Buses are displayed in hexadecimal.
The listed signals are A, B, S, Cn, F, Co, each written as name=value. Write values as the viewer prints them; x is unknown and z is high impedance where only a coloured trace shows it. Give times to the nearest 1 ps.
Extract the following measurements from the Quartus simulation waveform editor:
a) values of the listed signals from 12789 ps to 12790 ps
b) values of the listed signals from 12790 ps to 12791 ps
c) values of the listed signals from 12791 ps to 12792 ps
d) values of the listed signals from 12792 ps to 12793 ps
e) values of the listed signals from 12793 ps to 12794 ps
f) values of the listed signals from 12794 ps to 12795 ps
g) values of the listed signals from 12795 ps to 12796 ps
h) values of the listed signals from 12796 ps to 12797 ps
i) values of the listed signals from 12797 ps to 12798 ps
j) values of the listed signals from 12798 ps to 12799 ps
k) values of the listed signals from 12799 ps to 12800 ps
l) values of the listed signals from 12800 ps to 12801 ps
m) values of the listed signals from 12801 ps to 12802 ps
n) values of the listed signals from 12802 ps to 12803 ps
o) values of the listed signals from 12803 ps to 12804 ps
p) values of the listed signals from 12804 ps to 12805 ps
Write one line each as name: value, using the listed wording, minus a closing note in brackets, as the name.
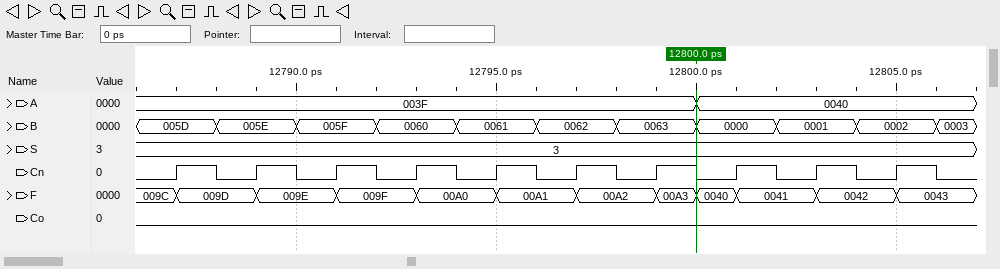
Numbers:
values of the listed signals from 12789 ps to 12790 ps: A=003F, B=005E, S=3, Cn=1, F=009E, Co=0
values of the listed signals from 12790 ps to 12791 ps: A=003F, B=005F, S=3, Cn=0, F=009E, Co=0
values of the listed signals from 12791 ps to 12792 ps: A=003F, B=005F, S=3, Cn=1, F=009F, Co=0
values of the listed signals from 12792 ps to 12793 ps: A=003F, B=0060, S=3, Cn=0, F=009F, Co=0
values of the listed signals from 12793 ps to 12794 ps: A=003F, B=0060, S=3, Cn=1, F=00A0, Co=0
values of the listed signals from 12794 ps to 12795 ps: A=003F, B=0061, S=3, Cn=0, F=00A0, Co=0
values of the listed signals from 12795 ps to 12796 ps: A=003F, B=0061, S=3, Cn=1, F=00A1, Co=0
values of the listed signals from 12796 ps to 12797 ps: A=003F, B=0062, S=3, Cn=0, F=00A1, Co=0
values of the listed signals from 12797 ps to 12798 ps: A=003F, B=0062, S=3, Cn=1, F=00A2, Co=0
values of the listed signals from 12798 ps to 12799 ps: A=003F, B=0063, S=3, Cn=0, F=00A2, Co=0
values of the listed signals from 12799 ps to 12800 ps: A=003F, B=0063, S=3, Cn=1, F=00A3, Co=0
values of the listed signals from 12800 ps to 12801 ps: A=0040, B=0000, S=3, Cn=0, F=0040, Co=0
values of the listed signals from 12801 ps to 12802 ps: A=0040, B=0000, S=3, Cn=1, F=0041, Co=0
values of the listed signals from 12802 ps to 12803 ps: A=0040, B=0001, S=3, Cn=0, F=0041, Co=0
values of the listed signals from 12803 ps to 12804 ps: A=0040, B=0001, S=3, Cn=1, F=0042, Co=0
values of the listed signals from 12804 ps to 12805 ps: A=0040, B=0002, S=3, Cn=0, F=0042, Co=0
